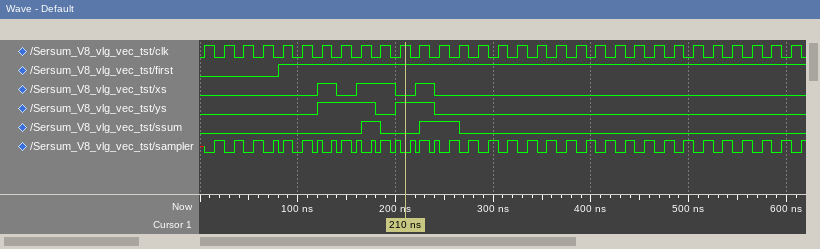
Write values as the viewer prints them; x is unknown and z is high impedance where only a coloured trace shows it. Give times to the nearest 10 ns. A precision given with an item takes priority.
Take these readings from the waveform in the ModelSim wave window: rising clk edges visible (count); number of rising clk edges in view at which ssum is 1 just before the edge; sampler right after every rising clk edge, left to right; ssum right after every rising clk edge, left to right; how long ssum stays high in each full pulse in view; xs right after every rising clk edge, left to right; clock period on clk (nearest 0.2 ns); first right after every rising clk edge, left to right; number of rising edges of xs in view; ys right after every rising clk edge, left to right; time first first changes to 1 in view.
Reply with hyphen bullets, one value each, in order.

- 31
- 3
- 0 0 0 0 1 1 0 1 0 1 0 1 0 0 0 0 0 0 0 0 0 0 0 0 0 0 0 0 0 0 0
- 0 0 0 0 0 0 0 0 1 0 0 1 1 0 0 0 0 0 0 0 0 0 0 0 0 0 0 0 0 0 0
- 20 ns, 40 ns
- 0 0 0 0 0 0 1 0 1 1 0 1 0 0 0 0 0 0 0 0 0 0 0 0 0 0 0 0 0 0 0
- 20 ns
- 0 0 0 0 1 1 1 1 1 1 1 1 1 1 1 1 1 1 1 1 1 1 1 1 1 1 1 1 1 1 1
- 3
- 0 0 0 0 0 0 1 1 1 0 1 1 0 0 0 0 0 0 0 0 0 0 0 0 0 0 0 0 0 0 0
- 80 ns
